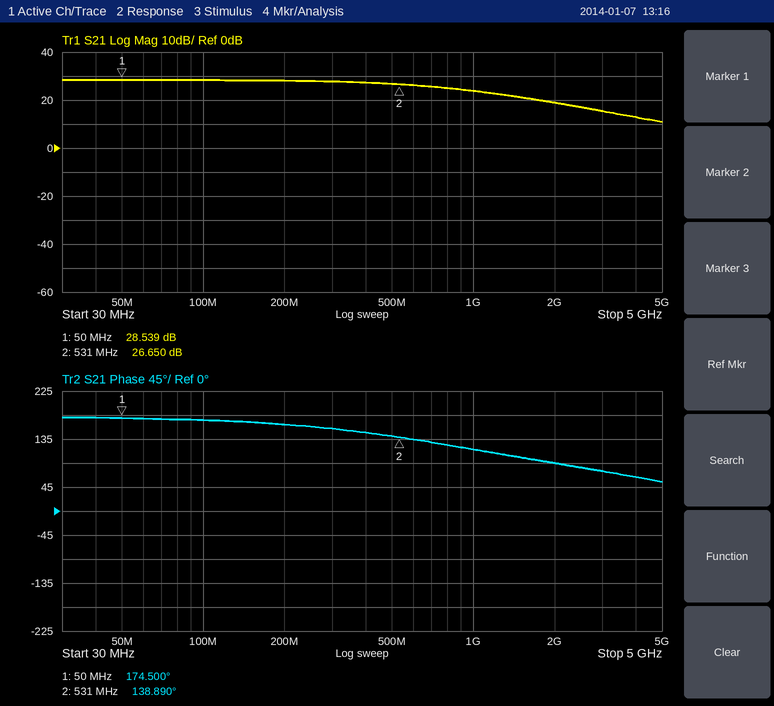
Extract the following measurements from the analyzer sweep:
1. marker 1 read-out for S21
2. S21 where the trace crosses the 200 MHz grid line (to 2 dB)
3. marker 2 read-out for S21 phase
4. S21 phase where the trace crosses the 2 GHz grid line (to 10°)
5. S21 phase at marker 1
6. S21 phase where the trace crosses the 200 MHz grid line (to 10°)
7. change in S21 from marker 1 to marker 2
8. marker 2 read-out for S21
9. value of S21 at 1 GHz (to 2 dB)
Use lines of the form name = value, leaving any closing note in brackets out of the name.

marker 1 read-out for S21 = 28.539 dB
S21 where the trace crosses the 200 MHz grid line = 28 dB
marker 2 read-out for S21 phase = 138.890°
S21 phase where the trace crosses the 2 GHz grid line = 90°
S21 phase at marker 1 = 174.500°
S21 phase where the trace crosses the 200 MHz grid line = 160°
change in S21 from marker 1 to marker 2 = -1.889 dB
marker 2 read-out for S21 = 26.650 dB
value of S21 at 1 GHz = 24 dB
